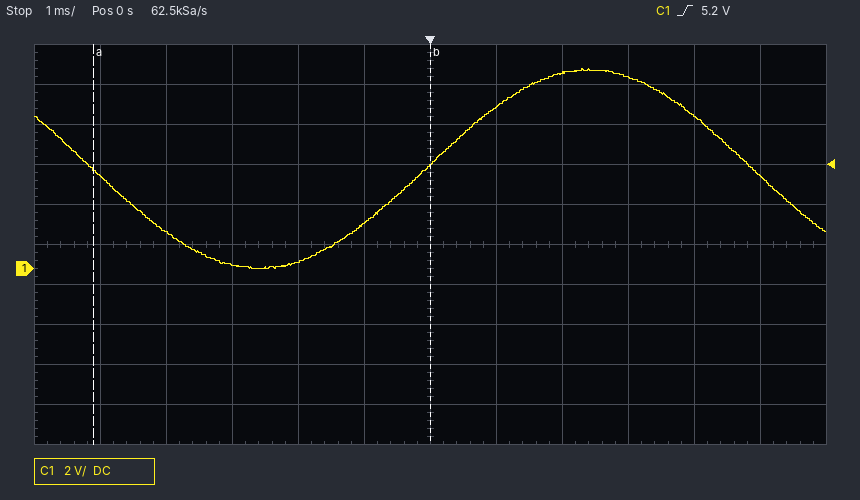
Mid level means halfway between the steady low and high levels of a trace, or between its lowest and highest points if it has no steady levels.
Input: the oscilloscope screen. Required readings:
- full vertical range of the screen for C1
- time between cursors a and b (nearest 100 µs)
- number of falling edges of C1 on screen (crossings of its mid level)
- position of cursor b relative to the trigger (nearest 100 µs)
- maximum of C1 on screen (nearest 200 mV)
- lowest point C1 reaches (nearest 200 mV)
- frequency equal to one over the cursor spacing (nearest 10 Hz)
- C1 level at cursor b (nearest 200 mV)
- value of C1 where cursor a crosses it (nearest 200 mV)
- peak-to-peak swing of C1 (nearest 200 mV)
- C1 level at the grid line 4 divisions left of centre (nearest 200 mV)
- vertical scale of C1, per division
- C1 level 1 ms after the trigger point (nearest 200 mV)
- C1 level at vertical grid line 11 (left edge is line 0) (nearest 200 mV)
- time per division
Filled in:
20 V
5.1 ms
2
0.0 ms
10.0 V
0.0 V
200 Hz
5.2 V
5.0 V
10.0 V
1.8 V
2 V
8.0 V
4.6 V
1 ms
